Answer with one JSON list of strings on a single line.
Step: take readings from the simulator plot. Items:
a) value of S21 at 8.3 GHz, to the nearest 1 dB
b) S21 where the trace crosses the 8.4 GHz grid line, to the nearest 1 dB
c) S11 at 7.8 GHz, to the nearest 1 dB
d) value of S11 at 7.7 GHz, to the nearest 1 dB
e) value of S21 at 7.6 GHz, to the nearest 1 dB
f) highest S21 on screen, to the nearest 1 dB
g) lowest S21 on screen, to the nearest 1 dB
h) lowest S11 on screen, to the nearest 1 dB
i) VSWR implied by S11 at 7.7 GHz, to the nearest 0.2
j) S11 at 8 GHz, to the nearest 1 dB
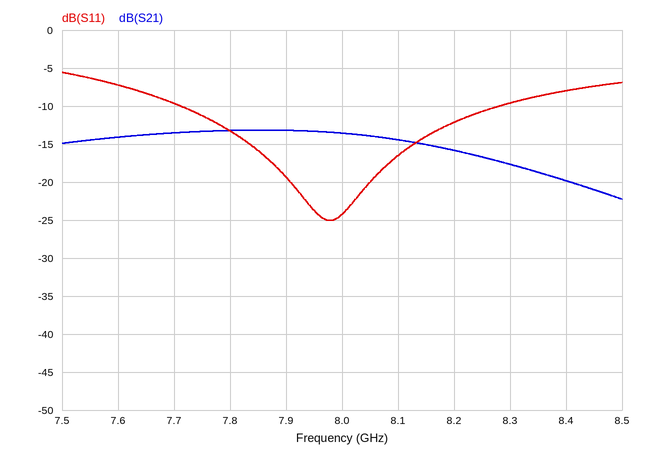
["-18 dB", "-20 dB", "-13 dB", "-10 dB", "-14 dB", "-13 dB", "-22 dB", "-25 dB", "2.0", "-24 dB"]
